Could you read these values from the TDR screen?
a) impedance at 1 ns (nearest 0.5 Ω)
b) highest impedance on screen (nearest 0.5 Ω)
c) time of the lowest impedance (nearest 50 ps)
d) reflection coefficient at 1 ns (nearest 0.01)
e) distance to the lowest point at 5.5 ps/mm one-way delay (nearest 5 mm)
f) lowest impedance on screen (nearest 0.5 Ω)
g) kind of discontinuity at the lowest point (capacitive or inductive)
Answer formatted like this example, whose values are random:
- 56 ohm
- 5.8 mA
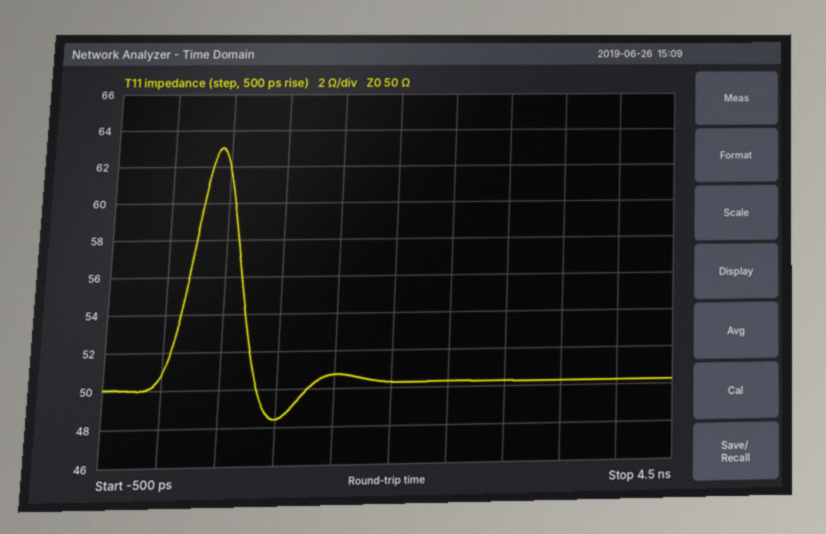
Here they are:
- 48.5 Ω
- 63.0 Ω
- 1.00 ns
- -0.02
- 90 mm
- 48.5 Ω
- capacitive
